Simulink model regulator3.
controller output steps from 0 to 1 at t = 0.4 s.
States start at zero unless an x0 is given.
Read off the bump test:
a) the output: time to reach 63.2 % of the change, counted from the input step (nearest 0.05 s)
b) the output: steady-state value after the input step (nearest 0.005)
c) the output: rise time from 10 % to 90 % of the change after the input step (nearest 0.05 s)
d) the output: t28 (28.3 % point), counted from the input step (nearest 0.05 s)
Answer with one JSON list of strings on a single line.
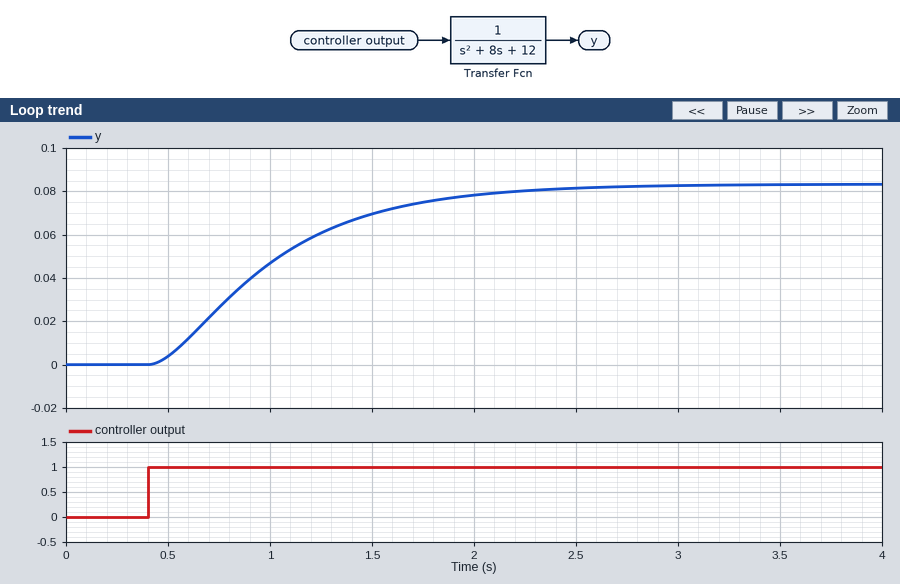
["0.70 s", "0.085", "1.20 s", "0.30 s"]
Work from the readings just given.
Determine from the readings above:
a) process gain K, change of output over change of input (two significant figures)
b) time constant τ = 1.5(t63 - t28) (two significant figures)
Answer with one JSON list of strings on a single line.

["0.085", "0.60 s"]
